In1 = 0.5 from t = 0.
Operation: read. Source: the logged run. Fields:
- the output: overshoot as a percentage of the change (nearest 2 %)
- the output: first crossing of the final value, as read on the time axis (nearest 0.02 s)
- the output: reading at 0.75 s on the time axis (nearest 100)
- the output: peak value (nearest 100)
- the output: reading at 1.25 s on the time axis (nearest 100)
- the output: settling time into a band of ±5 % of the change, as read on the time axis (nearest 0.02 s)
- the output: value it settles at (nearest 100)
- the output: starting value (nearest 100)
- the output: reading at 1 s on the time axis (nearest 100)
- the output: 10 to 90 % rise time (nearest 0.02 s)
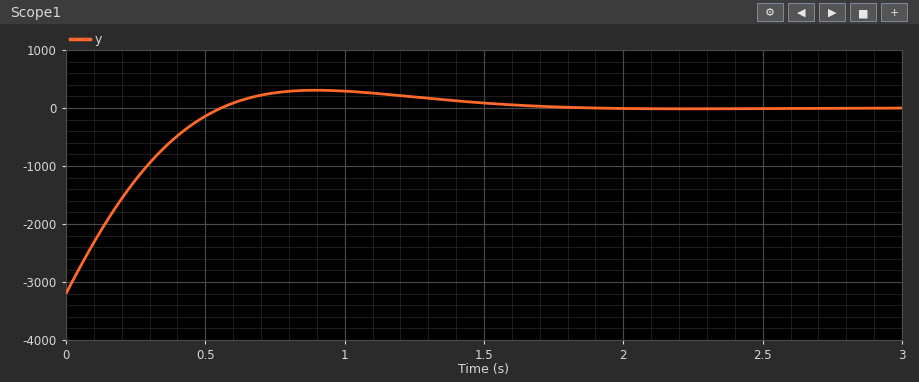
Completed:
10 %
0.56 s
300
300
200
1.32 s
0
-3200
300
0.40 s
